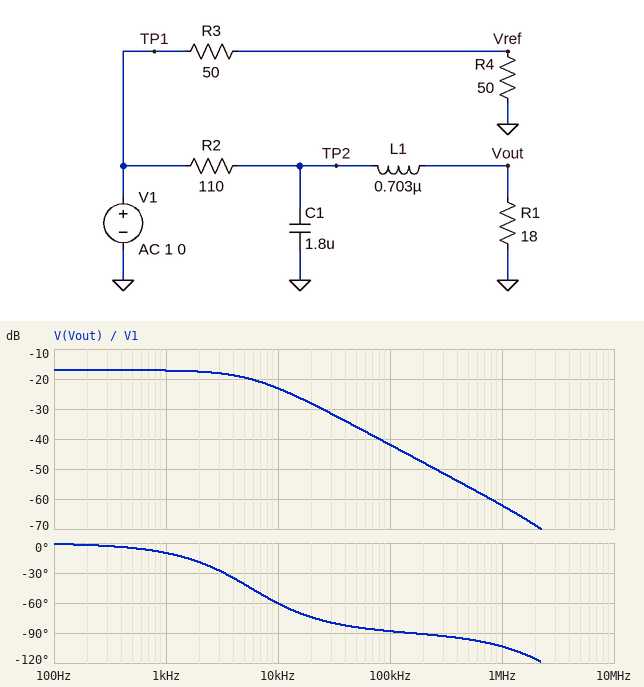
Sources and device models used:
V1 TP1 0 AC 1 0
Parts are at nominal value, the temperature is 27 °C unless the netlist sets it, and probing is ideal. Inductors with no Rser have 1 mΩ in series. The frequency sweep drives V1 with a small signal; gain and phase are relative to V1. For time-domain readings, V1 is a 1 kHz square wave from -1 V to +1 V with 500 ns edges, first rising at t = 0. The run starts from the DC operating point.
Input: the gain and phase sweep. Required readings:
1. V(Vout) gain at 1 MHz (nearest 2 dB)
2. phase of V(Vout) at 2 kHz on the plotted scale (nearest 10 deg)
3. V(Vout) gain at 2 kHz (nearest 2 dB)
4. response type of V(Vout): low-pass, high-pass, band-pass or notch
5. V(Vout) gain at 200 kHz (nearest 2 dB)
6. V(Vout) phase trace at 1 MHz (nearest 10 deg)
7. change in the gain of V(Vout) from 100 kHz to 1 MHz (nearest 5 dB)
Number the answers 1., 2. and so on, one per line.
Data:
1. -62 dB
2. -20 deg
3. -18 dB
4. low-pass
5. -48 dB
6. -100 deg
7. -20 dB
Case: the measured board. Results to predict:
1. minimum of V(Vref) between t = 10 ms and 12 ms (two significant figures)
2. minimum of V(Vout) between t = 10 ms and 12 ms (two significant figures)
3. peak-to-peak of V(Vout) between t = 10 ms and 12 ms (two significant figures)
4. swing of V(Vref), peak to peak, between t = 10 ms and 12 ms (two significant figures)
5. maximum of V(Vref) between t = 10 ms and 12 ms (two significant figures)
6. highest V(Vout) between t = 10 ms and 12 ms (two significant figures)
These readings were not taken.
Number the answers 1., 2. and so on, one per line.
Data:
1. -500 mV
2. -140 mV
3. 280 mV
4. 1.0 V
5. 500 mV
6. 140 mV
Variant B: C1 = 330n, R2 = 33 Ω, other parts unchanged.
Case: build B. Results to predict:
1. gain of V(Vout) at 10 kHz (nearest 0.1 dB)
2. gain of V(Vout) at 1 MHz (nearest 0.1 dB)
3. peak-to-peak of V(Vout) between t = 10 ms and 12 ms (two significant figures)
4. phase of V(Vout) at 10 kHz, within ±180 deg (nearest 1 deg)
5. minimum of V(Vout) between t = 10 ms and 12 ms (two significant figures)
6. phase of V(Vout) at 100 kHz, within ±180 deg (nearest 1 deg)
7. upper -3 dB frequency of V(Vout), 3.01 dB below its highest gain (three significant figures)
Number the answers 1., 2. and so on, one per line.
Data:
1. -9.3 dB
2. -36.9 dB
3. 710 mV
4. -14 deg
5. -350 mV
6. -69 deg
7. 41.7 kHz
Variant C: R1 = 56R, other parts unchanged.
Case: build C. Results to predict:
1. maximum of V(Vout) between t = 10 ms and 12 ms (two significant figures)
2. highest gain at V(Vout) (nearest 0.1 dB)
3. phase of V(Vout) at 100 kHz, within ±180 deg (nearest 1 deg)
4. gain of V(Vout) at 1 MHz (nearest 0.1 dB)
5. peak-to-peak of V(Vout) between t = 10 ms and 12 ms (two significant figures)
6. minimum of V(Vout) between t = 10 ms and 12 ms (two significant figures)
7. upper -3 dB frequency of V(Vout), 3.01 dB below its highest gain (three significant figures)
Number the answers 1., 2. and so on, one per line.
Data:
1. 340 mV
2. -9.4 dB
3. -89 deg
4. -61.9 dB
5. 670 mV
6. -340 mV
7. 2.38 kHz
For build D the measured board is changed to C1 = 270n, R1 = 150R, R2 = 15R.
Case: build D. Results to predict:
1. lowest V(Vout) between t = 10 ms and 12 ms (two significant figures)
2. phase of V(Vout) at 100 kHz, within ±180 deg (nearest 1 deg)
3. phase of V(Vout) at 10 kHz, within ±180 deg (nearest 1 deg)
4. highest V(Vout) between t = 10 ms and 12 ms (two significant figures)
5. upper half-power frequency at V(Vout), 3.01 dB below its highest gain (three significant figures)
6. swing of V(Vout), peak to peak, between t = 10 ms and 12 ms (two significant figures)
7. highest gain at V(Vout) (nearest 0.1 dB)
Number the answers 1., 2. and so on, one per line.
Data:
1. -910 mV
2. -67 deg
3. -13 deg
4. 910 mV
5. 43.2 kHz
6. 1.8 V
7. -0.8 dB
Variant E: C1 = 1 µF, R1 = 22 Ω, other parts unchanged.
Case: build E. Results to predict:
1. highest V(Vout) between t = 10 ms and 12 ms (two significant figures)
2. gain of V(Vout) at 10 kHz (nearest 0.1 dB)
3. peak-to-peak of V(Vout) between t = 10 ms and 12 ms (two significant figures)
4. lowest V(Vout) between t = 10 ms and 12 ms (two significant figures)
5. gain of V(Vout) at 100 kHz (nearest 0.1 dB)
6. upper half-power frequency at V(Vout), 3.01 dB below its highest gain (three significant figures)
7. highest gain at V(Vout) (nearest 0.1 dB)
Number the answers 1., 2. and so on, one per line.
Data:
1. 170 mV
2. -19.2 dB
3. 330 mV
4. -170 mV
5. -36.8 dB
6. 8.69 kHz
7. -15.6 dB
